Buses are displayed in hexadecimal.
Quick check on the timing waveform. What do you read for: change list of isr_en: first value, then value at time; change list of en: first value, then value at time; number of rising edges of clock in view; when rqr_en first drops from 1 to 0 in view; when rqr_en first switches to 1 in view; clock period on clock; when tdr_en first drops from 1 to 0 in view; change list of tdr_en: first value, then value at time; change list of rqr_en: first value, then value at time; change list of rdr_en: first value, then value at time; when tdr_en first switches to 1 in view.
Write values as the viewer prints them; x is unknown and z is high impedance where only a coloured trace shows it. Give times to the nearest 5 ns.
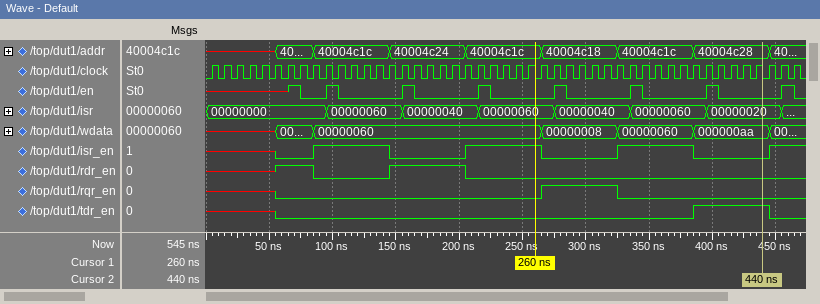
x, 0 at 55 ns, 1 at 85 ns, 0 at 145 ns, 1 at 205 ns, 0 at 265 ns, 1 at 325 ns, 0 at 385 ns, 1 at 445 ns
x, 1 at 65 ns, 0 at 75 ns, 1 at 95 ns, 0 at 105 ns, 1 at 155 ns, 0 at 165 ns, 1 at 215 ns, 0 at 225 ns, 1 at 275 ns, 0 at 285 ns, 1 at 335 ns, 0 at 345 ns, 1 at 395 ns, 0 at 405 ns, 1 at 455 ns, 0 at 465 ns
47
325 ns
265 ns
10 ns
445 ns
x, 0 at 55 ns, 1 at 385 ns, 0 at 445 ns
x, 0 at 55 ns, 1 at 265 ns, 0 at 325 ns
x, 1 at 55 ns, 0 at 85 ns, 1 at 145 ns, 0 at 205 ns
385 ns
